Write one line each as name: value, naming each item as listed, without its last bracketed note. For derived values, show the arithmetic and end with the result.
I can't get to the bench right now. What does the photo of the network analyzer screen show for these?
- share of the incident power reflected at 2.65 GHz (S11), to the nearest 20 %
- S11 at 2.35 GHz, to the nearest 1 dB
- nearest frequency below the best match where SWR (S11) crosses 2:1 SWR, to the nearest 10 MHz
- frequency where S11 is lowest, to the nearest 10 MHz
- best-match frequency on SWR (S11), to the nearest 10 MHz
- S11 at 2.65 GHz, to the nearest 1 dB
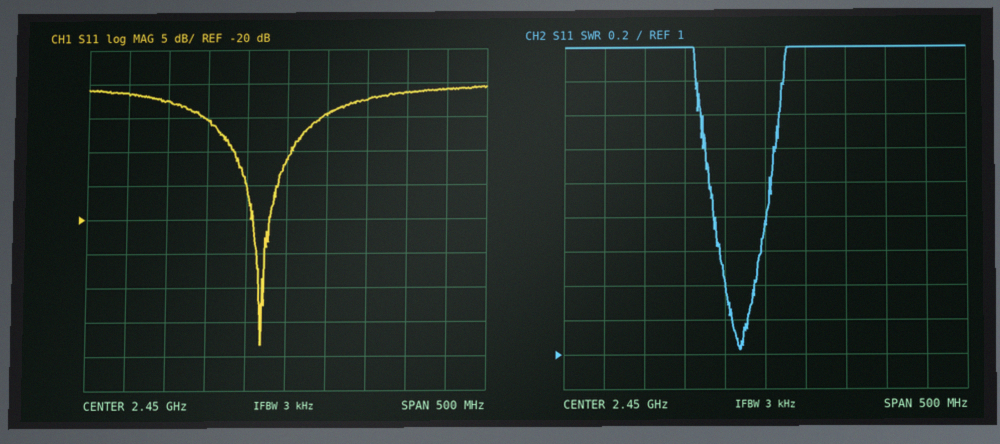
share of the incident power reflected at 2.65 GHz (S11), to the nearest 20 %: 10^(-1/10) ≈ 79.4 %, so 80 % to the nearest 20 %
S11 at 2.35 GHz, to the nearest 1 dB: -5 dB
nearest frequency below the best match where SWR (S11) crosses 2:1 SWR, to the nearest 10 MHz: 2.38 GHz
frequency where S11 is lowest, to the nearest 10 MHz: 2.42 GHz
best-match frequency on SWR (S11), to the nearest 10 MHz: 2.42 GHz
S11 at 2.65 GHz, to the nearest 1 dB: -1 dB
